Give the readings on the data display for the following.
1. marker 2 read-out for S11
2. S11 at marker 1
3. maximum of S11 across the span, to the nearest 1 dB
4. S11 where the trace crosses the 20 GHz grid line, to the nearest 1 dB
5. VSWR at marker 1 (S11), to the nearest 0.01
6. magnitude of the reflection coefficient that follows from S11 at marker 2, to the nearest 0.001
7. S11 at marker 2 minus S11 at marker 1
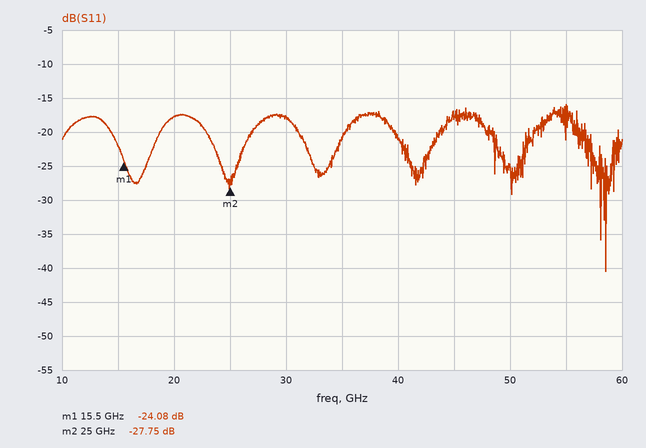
-27.75 dB
-24.08 dB
-16 dB
-18 dB
1.13
0.041
-3.67 dB
